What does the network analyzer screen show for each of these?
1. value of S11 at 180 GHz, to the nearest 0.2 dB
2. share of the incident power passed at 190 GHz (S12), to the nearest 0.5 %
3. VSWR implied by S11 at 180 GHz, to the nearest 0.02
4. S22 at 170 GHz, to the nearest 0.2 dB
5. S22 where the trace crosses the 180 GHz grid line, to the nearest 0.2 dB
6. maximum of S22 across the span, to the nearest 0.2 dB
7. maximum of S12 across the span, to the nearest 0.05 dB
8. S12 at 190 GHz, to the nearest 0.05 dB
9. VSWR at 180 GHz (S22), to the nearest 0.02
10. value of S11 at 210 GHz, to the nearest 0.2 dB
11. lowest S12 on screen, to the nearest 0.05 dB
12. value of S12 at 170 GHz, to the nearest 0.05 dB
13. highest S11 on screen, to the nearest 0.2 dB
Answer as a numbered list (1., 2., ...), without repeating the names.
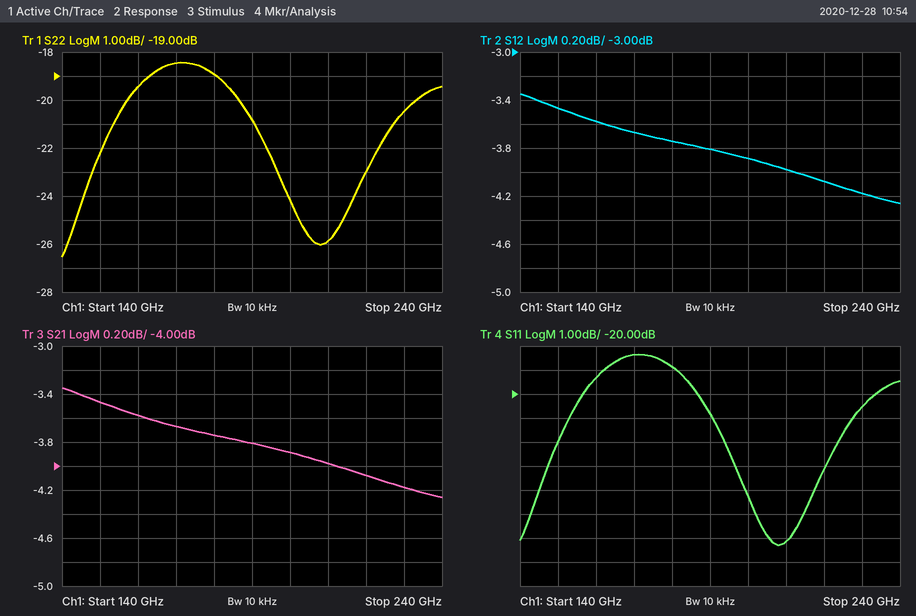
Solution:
1. -18.8 dB
2. 41.5 %
3. 1.26
4. -18.4 dB
5. -19.0 dB
6. -18.4 dB
7. -3.35 dB
8. -3.80 dB
9. 1.26
10. -26.2 dB
11. -4.25 dB
12. -3.65 dB
13. -18.4 dB
